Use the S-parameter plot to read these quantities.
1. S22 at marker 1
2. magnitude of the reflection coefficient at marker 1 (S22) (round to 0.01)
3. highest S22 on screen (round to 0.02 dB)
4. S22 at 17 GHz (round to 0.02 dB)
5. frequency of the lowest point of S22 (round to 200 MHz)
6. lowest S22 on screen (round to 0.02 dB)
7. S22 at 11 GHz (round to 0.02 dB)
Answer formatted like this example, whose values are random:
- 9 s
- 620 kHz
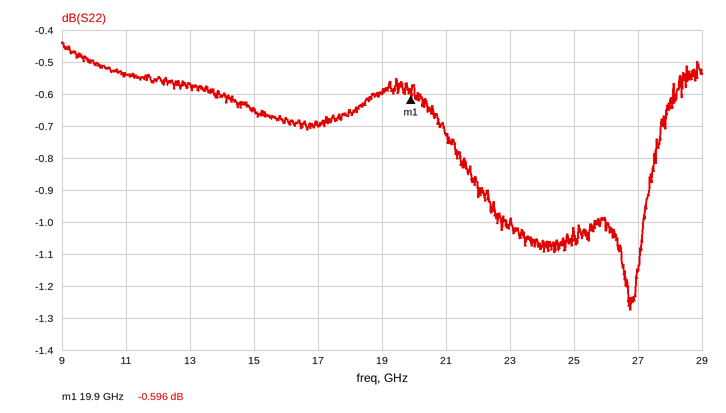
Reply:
- -0.596 dB
- 0.93
- -0.44 dB
- -0.70 dB
- 26.8 GHz
- -1.28 dB
- -0.54 dB
